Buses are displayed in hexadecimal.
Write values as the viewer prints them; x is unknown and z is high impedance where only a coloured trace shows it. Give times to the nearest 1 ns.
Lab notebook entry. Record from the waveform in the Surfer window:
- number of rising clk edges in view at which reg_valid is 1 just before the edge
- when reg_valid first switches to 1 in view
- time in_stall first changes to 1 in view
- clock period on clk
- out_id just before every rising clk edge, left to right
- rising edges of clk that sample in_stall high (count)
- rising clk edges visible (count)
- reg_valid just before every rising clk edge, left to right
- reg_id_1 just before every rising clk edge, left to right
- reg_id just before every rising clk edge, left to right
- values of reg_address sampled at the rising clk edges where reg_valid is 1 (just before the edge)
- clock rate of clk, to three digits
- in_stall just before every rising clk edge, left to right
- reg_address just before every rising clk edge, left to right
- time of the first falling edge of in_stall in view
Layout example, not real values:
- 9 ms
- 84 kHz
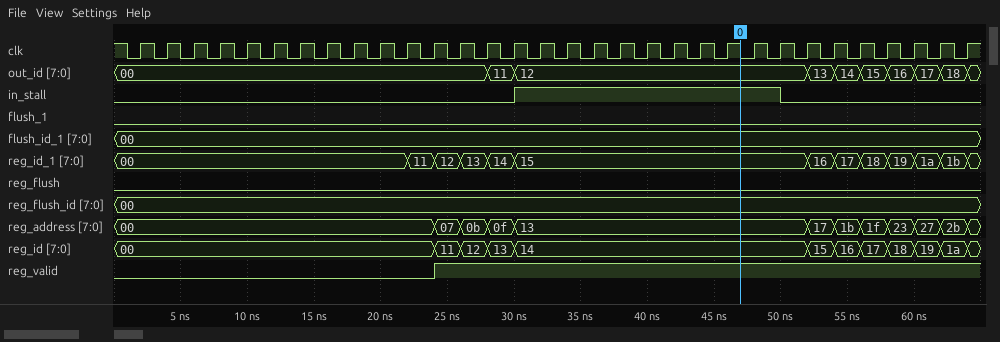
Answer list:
- 20
- 24 ns
- 30 ns
- 2 ns
- 00, 00, 00, 00, 00, 00, 00, 00, 00, 00, 00, 00, 00, 00, 11, 12, 12, 12, 12, 12, 12, 12, 12, 12, 12, 12, 13, 14, 15, 16, 17, 18
- 10
- 32
- 0 0 0 0 0 0 0 0 0 0 0 0 1 1 1 1 1 1 1 1 1 1 1 1 1 1 1 1 1 1 1 1
- 00, 00, 00, 00, 00, 00, 00, 00, 00, 00, 00, 11, 12, 13, 14, 15, 15, 15, 15, 15, 15, 15, 15, 15, 15, 15, 16, 17, 18, 19, 1a, 1b
- 00, 00, 00, 00, 00, 00, 00, 00, 00, 00, 00, 00, 11, 12, 13, 14, 14, 14, 14, 14, 14, 14, 14, 14, 14, 14, 15, 16, 17, 18, 19, 1a
- 07, 0b, 0f, 13, 13, 13, 13, 13, 13, 13, 13, 13, 13, 13, 17, 1b, 1f, 23, 27, 2b
- 500 MHz
- 0 0 0 0 0 0 0 0 0 0 0 0 0 0 0 1 1 1 1 1 1 1 1 1 1 0 0 0 0 0 0 0
- 00, 00, 00, 00, 00, 00, 00, 00, 00, 00, 00, 00, 07, 0b, 0f, 13, 13, 13, 13, 13, 13, 13, 13, 13, 13, 13, 17, 1b, 1f, 23, 27, 2b
- 50 ns
